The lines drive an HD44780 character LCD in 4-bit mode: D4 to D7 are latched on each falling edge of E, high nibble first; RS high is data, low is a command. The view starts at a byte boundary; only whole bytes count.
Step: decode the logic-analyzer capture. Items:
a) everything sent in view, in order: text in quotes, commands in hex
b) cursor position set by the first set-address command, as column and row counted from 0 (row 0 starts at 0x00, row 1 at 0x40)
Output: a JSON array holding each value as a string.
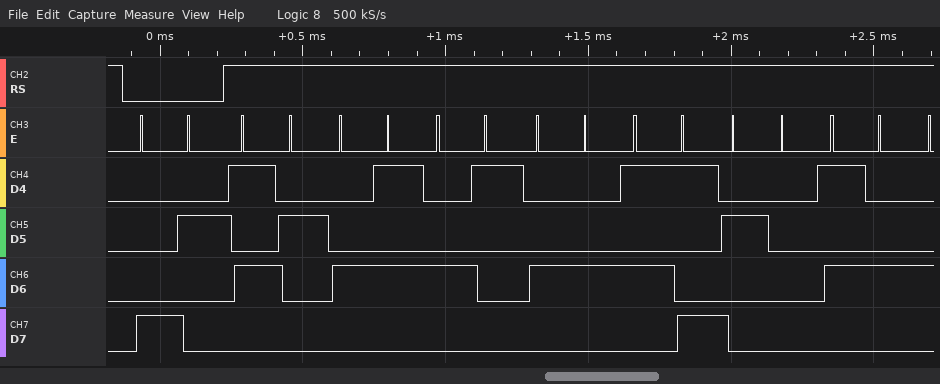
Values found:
["0x82 \"READY T\"", "column 2, row 0"]
